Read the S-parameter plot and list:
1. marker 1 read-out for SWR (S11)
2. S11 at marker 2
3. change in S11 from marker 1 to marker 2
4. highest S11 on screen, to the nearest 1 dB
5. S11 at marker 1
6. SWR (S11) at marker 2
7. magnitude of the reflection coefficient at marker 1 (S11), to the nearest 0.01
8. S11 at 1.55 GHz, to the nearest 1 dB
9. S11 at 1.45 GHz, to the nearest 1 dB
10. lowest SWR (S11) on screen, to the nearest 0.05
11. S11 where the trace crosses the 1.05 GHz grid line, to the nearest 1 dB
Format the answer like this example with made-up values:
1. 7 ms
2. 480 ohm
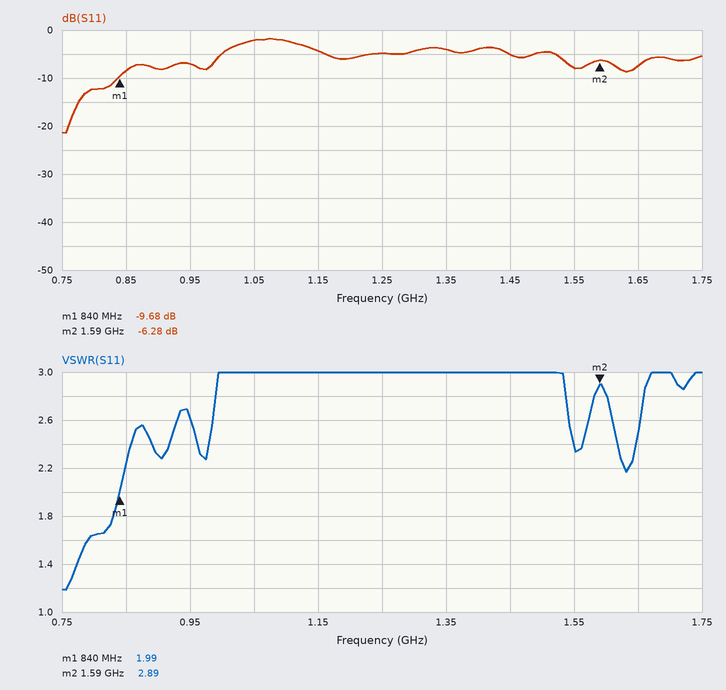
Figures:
1. 1.99
2. -6.28 dB
3. 3.40 dB
4. -2 dB
5. -9.68 dB
6. 2.89
7. 0.33
8. -8 dB
9. -5 dB
10. 1.20
11. -2 dB
